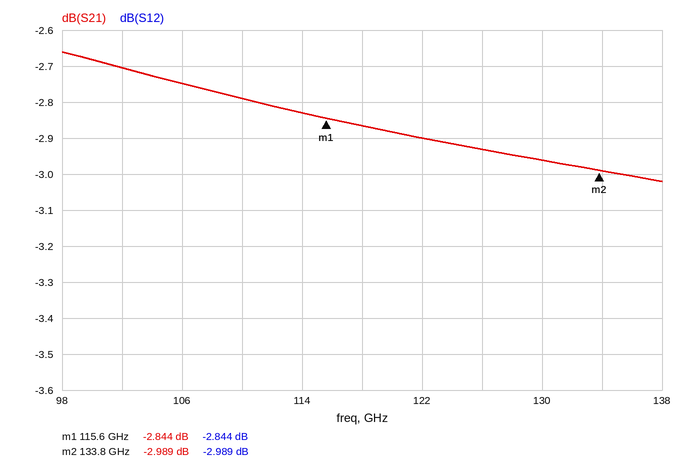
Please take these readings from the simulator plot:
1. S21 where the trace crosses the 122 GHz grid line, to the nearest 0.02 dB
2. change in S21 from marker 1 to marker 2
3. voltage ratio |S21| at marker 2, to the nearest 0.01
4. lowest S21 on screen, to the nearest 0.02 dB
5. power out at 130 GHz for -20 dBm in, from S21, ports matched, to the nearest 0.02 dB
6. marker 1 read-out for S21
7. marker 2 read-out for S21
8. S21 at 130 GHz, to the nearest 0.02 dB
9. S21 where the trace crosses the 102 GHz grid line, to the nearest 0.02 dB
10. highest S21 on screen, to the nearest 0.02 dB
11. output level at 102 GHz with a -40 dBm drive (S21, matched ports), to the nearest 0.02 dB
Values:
-2.90 dB
-0.145 dB
0.71
-3.02 dB
-22.96 dBm
-2.844 dB
-2.989 dB
-2.96 dB
-2.70 dB
-2.66 dB
-42.70 dBm
